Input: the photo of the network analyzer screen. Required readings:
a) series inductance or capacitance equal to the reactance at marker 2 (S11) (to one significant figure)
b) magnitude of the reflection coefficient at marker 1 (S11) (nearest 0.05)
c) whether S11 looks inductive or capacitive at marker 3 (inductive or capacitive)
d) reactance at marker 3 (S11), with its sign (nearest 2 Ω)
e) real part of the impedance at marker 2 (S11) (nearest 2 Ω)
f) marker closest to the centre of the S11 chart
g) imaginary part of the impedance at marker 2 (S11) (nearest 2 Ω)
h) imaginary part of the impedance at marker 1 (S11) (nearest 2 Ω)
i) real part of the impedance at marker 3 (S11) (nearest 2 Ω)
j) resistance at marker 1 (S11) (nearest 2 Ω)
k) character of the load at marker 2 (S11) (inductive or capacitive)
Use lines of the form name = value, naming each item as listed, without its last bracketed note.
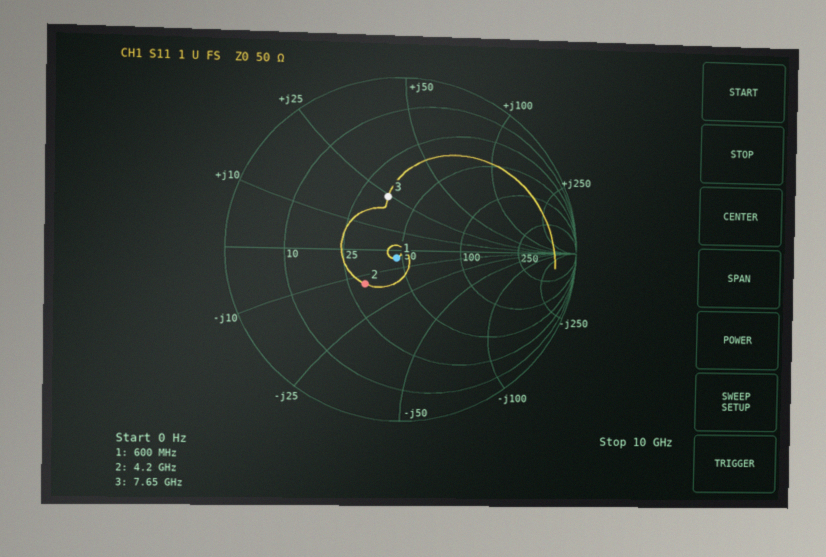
series inductance or capacitance equal to the reactance at marker 2 (S11) = 3 pF
magnitude of the reflection coefficient at marker 1 (S11) = 0.05
whether S11 looks inductive or capacitive at marker 3 = inductive
reactance at marker 3 (S11), with its sign = +24 Ω
real part of the impedance at marker 2 (S11) = 30 Ω
marker closest to the centre of the S11 chart = marker 1
imaginary part of the impedance at marker 2 (S11) = -14 Ω
imaginary part of the impedance at marker 1 (S11) = -4 Ω
real part of the impedance at marker 3 (S11) = 36 Ω
resistance at marker 1 (S11) = 46 Ω
character of the load at marker 2 (S11) = capacitive
